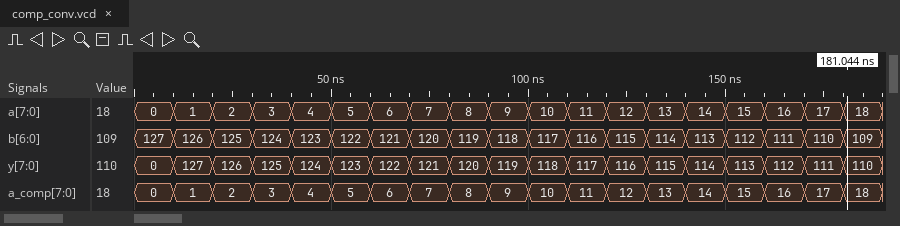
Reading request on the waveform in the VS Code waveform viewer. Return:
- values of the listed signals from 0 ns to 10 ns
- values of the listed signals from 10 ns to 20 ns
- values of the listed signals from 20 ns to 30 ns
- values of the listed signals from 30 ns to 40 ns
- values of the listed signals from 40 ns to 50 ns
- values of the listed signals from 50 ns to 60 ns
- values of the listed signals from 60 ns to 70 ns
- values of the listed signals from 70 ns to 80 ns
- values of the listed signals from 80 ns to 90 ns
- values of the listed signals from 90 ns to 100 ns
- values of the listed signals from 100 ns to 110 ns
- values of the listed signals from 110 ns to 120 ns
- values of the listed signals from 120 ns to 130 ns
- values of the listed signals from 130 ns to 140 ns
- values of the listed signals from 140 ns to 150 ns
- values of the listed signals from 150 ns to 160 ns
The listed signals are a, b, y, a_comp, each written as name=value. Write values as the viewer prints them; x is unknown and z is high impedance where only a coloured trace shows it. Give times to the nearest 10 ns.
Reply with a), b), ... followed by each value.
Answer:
a) a=0, b=127, y=0, a_comp=0
b) a=1, b=126, y=127, a_comp=1
c) a=2, b=125, y=126, a_comp=2
d) a=3, b=124, y=125, a_comp=3
e) a=4, b=123, y=124, a_comp=4
f) a=5, b=122, y=123, a_comp=5
g) a=6, b=121, y=122, a_comp=6
h) a=7, b=120, y=121, a_comp=7
i) a=8, b=119, y=120, a_comp=8
j) a=9, b=118, y=119, a_comp=9
k) a=10, b=117, y=118, a_comp=10
l) a=11, b=116, y=117, a_comp=11
m) a=12, b=115, y=116, a_comp=12
n) a=13, b=114, y=115, a_comp=13
o) a=14, b=113, y=114, a_comp=14
p) a=15, b=112, y=113, a_comp=15
